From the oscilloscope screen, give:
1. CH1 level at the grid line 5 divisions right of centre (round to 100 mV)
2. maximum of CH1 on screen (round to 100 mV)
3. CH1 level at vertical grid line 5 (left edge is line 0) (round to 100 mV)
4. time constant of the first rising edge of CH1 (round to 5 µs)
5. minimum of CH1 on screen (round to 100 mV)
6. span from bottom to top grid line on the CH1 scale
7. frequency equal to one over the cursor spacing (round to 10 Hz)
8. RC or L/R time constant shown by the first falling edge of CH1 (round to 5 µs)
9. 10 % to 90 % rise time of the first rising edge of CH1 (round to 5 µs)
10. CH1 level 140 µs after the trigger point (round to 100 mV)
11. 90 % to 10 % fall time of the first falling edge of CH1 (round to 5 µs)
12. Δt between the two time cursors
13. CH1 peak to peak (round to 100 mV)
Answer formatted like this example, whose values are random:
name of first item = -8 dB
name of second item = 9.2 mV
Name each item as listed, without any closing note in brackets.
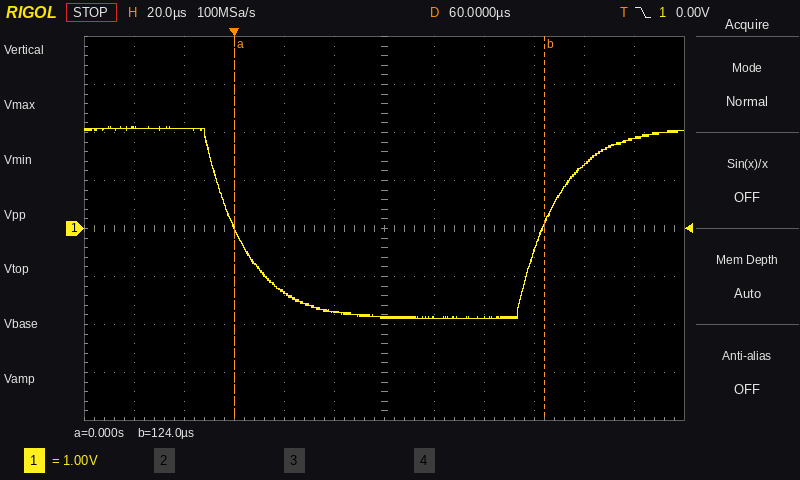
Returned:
CH1 level at the grid line 5 divisions right of centre = 1.9 V
maximum of CH1 on screen = 2.1 V
CH1 level at vertical grid line 5 (left edge is line 0) = -1.7 V
time constant of the first rising edge of CH1 = 15 µs
minimum of CH1 on screen = -1.9 V
span from bottom to top grid line on the CH1 scale = 8 V
frequency equal to one over the cursor spacing = 8.06 kHz
RC or L/R time constant shown by the first falling edge of CH1 = 15 µs
10 % to 90 % rise time of the first rising edge of CH1 = 35 µs
CH1 level 140 µs after the trigger point = 1.3 V
90 % to 10 % fall time of the first falling edge of CH1 = 35 µs
Δt between the two time cursors = 124 µs
CH1 peak to peak = 4.0 V
